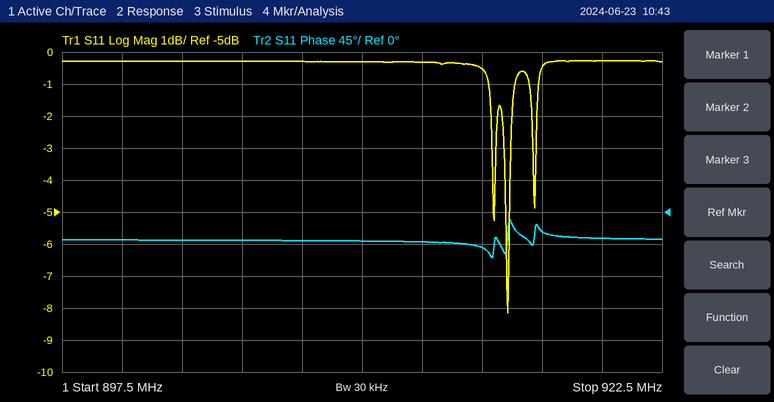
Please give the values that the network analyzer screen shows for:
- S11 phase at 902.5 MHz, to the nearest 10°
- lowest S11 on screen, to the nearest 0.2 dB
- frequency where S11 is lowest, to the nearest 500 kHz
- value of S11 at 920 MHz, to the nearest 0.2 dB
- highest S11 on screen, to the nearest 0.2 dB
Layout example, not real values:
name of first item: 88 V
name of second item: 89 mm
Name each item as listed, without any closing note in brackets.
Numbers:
S11 phase at 902.5 MHz, to the nearest 10°: -40°
lowest S11 on screen, to the nearest 0.2 dB: -8.2 dB
frequency where S11 is lowest, to the nearest 500 kHz: 916.0 MHz
value of S11 at 920 MHz, to the nearest 0.2 dB: -0.2 dB
highest S11 on screen, to the nearest 0.2 dB: -0.2 dB
